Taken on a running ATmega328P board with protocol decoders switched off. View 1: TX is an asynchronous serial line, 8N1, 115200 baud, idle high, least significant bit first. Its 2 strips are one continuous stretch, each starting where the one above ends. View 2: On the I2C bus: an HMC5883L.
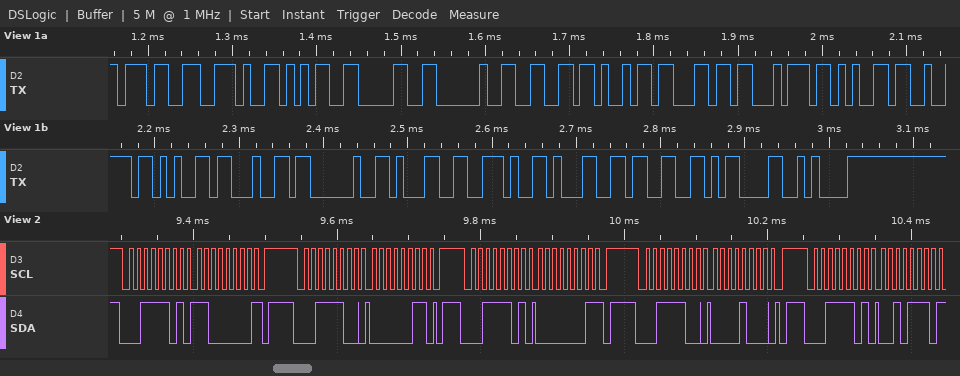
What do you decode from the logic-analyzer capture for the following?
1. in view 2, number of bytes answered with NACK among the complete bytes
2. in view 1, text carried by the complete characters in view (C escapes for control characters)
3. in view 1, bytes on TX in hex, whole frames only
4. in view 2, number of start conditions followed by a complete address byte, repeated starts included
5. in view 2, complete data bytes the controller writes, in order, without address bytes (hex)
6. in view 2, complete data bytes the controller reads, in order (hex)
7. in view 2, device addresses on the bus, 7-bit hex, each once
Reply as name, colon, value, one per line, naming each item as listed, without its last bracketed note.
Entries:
in view 2, number of bytes answered with NACK among the complete bytes: 3
in view 1, text carried by the complete characters in view: "7.50 filtered 1.13\r\n"
in view 1, bytes on TX in hex, whole frames only: 0x37 0x2E 0x35 0x30 0x20 0x66 0x69 0x6C 0x74 0x65 0x72 0x65 0x64 0x20 0x31 0x2E 0x31 0x33 0x0D 0x0A
in view 2, number of start conditions followed by a complete address byte, repeated starts included: 5
in view 2, complete data bytes the controller writes, in order, without address bytes: 03 08
in view 2, complete data bytes the controller reads, in order: C0 01 2E
in view 2, device addresses on the bus, 7-bit hex, each once: 0x1E
